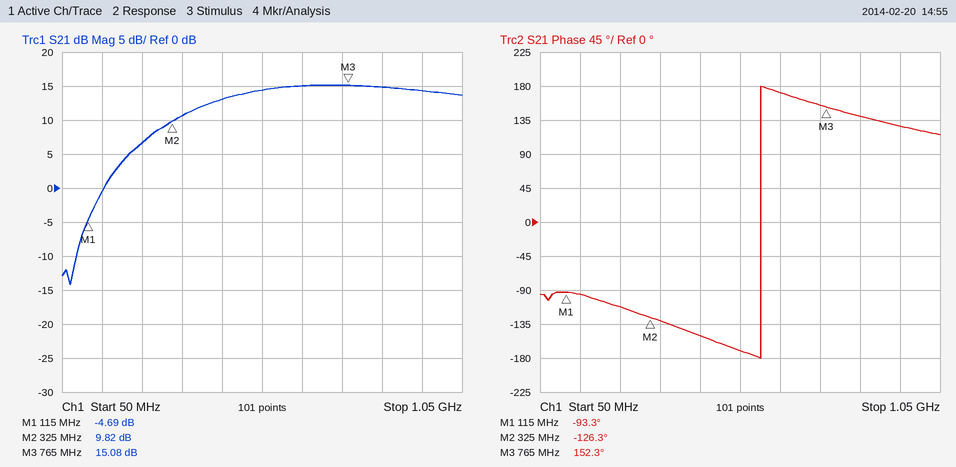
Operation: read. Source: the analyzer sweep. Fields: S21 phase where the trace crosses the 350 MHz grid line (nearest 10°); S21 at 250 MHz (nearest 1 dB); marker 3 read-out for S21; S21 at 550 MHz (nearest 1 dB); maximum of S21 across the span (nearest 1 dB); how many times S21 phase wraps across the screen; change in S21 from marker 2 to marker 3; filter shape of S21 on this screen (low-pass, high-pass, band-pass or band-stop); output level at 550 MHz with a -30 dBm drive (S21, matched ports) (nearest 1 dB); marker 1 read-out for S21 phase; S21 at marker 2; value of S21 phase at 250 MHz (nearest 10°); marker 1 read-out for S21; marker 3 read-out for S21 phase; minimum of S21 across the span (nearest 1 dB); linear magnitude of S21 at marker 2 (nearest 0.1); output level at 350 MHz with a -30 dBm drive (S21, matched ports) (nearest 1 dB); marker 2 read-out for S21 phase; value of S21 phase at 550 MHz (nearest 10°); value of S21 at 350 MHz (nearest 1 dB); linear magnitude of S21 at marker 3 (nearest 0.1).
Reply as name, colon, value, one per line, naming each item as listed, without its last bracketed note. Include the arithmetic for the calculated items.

S21 phase where the trace crosses the 350 MHz grid line: -130°
S21 at 250 MHz: 7 dB
marker 3 read-out for S21: 15.08 dB
S21 at 550 MHz: 14 dB
maximum of S21 across the span: 15 dB
how many times S21 phase wraps across the screen: 1
change in S21 from marker 2 to marker 3: 15.08 − (9.82) = 5.26 dB
filter shape of S21 on this screen: high-pass
output level at 550 MHz with a -30 dBm drive (S21, matched ports): -30 dBm + (14 dB) = -16 dBm
marker 1 read-out for S21 phase: -93.3°
S21 at marker 2: 9.82 dB
value of S21 phase at 250 MHz: -110°
marker 1 read-out for S21: -4.69 dB
marker 3 read-out for S21 phase: 152.3°
minimum of S21 across the span: -14 dB
linear magnitude of S21 at marker 2: 10^(9.82/20) ≈ 3.1
output level at 350 MHz with a -30 dBm drive (S21, matched ports): -30 dBm + (11 dB) = -19 dBm
marker 2 read-out for S21 phase: -126.3°
value of S21 phase at 550 MHz: -170°
value of S21 at 350 MHz: 11 dB
linear magnitude of S21 at marker 3: 10^(15.08/20) ≈ 5.7
